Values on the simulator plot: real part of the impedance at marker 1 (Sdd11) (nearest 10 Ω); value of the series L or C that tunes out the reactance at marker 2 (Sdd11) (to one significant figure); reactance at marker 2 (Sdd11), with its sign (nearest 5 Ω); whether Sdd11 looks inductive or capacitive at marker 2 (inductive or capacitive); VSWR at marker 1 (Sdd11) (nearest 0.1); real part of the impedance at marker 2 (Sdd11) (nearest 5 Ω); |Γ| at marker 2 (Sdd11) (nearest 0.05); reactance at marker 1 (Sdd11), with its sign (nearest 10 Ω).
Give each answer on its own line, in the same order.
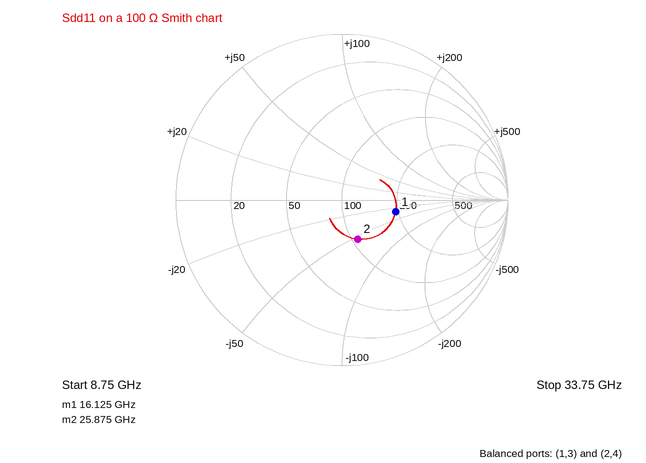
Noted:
190 Ω
300 pH
-55 Ω
capacitive
2.0
105 Ω
0.25
-30 Ω
